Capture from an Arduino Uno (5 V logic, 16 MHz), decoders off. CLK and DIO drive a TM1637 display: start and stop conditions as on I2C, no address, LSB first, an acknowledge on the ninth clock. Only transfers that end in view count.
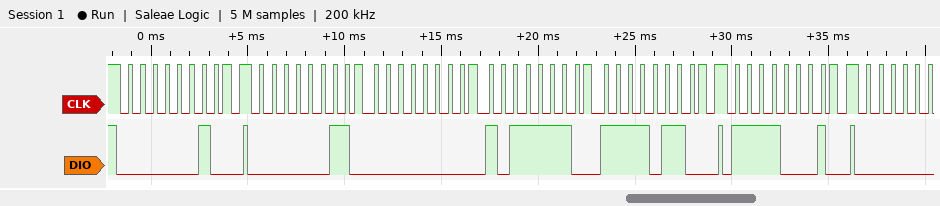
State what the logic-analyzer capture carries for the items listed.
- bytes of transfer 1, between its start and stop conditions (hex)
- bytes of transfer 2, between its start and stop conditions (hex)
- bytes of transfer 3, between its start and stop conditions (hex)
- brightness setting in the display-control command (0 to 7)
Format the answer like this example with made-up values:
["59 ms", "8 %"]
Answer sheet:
["40", "C0 00 7D 6F", "8F", "7"]
